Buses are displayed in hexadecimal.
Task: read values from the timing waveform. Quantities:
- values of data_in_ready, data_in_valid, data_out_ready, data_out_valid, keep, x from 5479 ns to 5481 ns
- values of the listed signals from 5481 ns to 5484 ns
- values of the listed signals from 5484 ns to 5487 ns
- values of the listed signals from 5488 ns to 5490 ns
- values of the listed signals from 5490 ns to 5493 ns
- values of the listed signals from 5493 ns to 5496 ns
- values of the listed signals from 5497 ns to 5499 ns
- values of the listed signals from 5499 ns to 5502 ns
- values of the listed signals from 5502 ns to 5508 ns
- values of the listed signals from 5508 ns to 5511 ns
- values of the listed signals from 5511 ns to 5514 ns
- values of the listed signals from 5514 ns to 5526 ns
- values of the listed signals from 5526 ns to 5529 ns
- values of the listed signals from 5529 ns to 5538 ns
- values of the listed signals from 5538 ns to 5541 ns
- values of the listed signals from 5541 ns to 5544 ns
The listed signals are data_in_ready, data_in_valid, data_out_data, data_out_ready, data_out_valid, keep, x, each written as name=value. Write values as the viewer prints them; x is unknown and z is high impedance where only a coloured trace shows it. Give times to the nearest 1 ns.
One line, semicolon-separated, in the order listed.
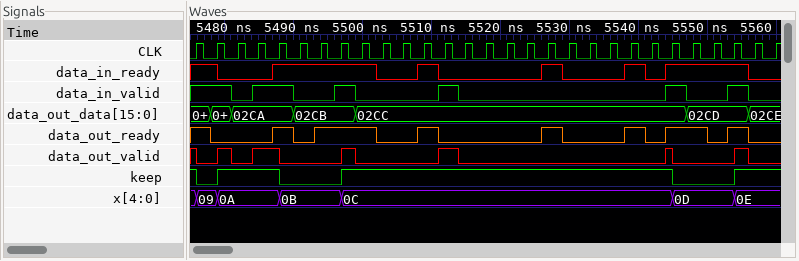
data_in_ready=0, data_in_valid=1, data_out_ready=0, data_out_valid=1, keep=1, x=0A; data_in_ready=0, data_in_valid=0, data_out_data=02CA, data_out_ready=0, data_out_valid=0, keep=1, x=0A; data_in_ready=0, data_in_valid=1, data_out_data=02CA, data_out_ready=0, data_out_valid=1, keep=1, x=0A; data_in_ready=1, data_in_valid=1, data_out_data=02CA, data_out_ready=1, data_out_valid=0, keep=0, x=0B; data_in_ready=1, data_in_valid=0, data_out_data=02CB, data_out_ready=0, data_out_valid=0, keep=0, x=0B; data_in_ready=1, data_in_valid=0, data_out_data=02CB, data_out_ready=1, data_out_valid=0, keep=0, x=0B; data_in_ready=1, data_in_valid=1, data_out_data=02CB, data_out_ready=1, data_out_valid=1, keep=1, x=0C; data_in_ready=1, data_in_valid=0, data_out_data=02CC, data_out_ready=1, data_out_valid=0, keep=1, x=0C; data_in_ready=0, data_in_valid=0, data_out_data=02CC, data_out_ready=0, data_out_valid=0, keep=1, x=0C; data_in_ready=1, data_in_valid=0, data_out_data=02CC, data_out_ready=1, data_out_valid=0, keep=1, x=0C; data_in_ready=0, data_in_valid=1, data_out_data=02CC, data_out_ready=0, data_out_valid=1, keep=1, x=0C; data_in_ready=0, data_in_valid=0, data_out_data=02CC, data_out_ready=0, data_out_valid=0, keep=1, x=0C; data_in_ready=1, data_in_valid=0, data_out_data=02CC, data_out_ready=1, data_out_valid=0, keep=1, x=0C; data_in_ready=0, data_in_valid=0, data_out_data=02CC, data_out_ready=0, data_out_valid=0, keep=1, x=0C; data_in_ready=1, data_in_valid=0, data_out_data=02CC, data_out_ready=1, data_out_valid=0, keep=1, x=0C; data_in_ready=0, data_in_valid=0, data_out_data=02CC, data_out_ready=0, data_out_valid=0, keep=1, x=0C
